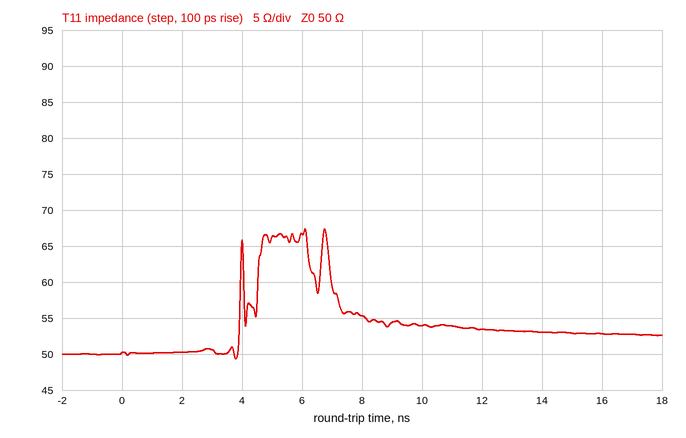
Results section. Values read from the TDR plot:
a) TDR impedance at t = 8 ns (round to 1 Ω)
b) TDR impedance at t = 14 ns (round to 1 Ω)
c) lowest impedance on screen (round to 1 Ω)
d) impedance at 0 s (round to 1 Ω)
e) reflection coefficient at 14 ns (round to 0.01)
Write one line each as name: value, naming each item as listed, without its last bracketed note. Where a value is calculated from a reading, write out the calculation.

TDR impedance at t = 8 ns: 55 Ω
TDR impedance at t = 14 ns: 53 Ω
lowest impedance on screen: 49 Ω
impedance at 0 s: 50 Ω
reflection coefficient at 14 ns: (53 − 50)/(53 + 50) ≈ +0.03
